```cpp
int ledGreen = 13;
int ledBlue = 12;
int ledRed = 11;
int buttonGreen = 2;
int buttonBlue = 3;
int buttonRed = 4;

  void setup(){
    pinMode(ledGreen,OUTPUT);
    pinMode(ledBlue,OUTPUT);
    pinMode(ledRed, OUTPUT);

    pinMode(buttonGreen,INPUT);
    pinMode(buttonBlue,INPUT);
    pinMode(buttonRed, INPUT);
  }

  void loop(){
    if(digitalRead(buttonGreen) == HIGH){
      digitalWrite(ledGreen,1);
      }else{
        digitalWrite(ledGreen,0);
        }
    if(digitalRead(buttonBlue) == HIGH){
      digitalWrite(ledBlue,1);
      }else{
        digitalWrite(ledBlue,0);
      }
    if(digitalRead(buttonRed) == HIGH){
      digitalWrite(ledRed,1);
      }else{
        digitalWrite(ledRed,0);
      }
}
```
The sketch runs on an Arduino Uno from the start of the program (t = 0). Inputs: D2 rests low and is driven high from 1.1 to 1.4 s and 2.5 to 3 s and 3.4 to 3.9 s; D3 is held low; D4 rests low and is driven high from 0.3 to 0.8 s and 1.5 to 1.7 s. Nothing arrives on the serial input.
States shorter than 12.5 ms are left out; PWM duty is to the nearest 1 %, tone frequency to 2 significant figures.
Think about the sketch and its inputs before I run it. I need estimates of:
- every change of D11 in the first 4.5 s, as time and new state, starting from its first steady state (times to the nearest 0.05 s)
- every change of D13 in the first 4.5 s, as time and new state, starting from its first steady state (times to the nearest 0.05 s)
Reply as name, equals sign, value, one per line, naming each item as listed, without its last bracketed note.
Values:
every change of D11 in the first 4.5 s, as time and new state, starting from its first steady state = 0 s low; 0.3 s high; 0.8 s low; 1.5 s high; 1.7 s low
every change of D13 in the first 4.5 s, as time and new state, starting from its first steady state = 0 s low; 1.1 s high; 1.4 s low; 2.5 s high; 3 s low; 3.4 s high; 3.9 s low
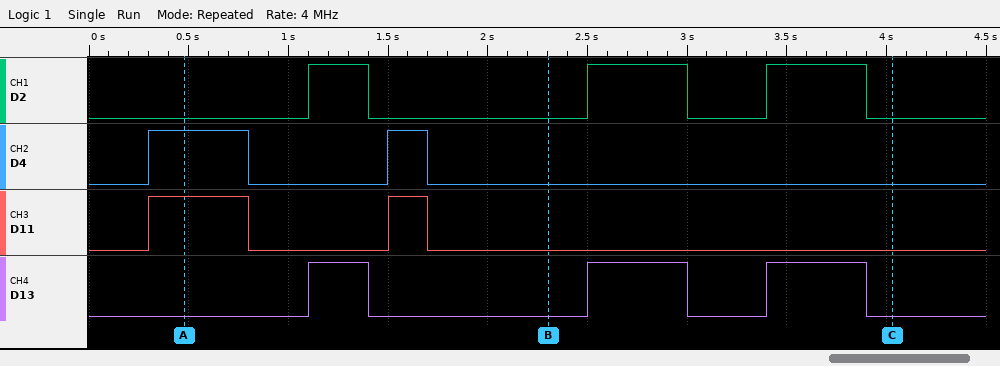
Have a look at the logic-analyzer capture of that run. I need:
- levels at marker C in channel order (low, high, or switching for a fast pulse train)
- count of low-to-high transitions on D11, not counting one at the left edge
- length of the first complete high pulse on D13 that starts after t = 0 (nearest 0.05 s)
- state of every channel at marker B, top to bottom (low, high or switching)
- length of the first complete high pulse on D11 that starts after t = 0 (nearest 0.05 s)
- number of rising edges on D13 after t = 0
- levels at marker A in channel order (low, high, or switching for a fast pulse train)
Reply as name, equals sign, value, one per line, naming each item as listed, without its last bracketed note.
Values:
levels at marker C in channel order = D2 low, D4 low, D11 low, D13 low
count of low-to-high transitions on D11, not counting one at the left edge = 2
length of the first complete high pulse on D13 that starts after t = 0 = 0.30 s
state of every channel at marker B, top to bottom = D2 low, D4 low, D11 low, D13 low
length of the first complete high pulse on D11 that starts after t = 0 = 0.50 s
number of rising edges on D13 after t = 0 = 3
levels at marker A in channel order = D2 low, D4 high, D11 high, D13 low
